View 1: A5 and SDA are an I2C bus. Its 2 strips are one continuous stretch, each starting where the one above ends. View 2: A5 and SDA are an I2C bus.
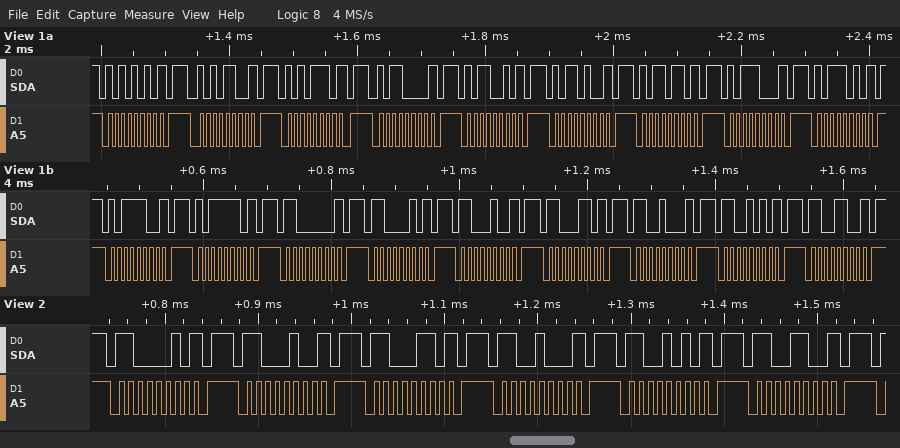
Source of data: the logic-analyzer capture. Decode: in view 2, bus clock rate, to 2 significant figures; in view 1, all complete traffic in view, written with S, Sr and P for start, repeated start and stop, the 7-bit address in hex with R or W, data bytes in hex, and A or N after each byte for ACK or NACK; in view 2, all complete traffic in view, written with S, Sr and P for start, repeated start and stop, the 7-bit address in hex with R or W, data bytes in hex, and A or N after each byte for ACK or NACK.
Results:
100 kHz
S 55W N P S 56W N P S 57W N P S 58W N P S 59W N P S 5AW N P S 5BW N P S 5CW N P S 5DW N P S 5EW N P S 5FW N P S 60W N P S 61W N P S 62W N P S 63W N P S 64W N P S 65W N P S 66W N P
S 61W N P S 62W N P S 63W N P S 64W N P S 65W N P S 66W N P
